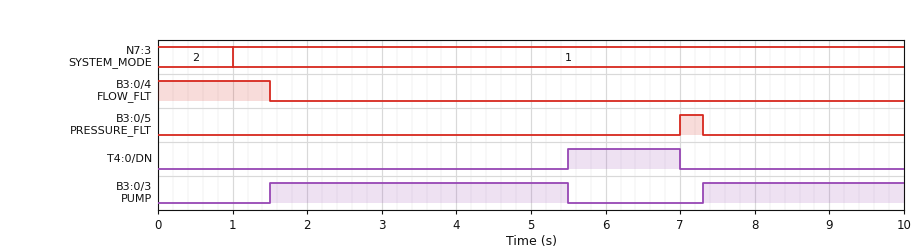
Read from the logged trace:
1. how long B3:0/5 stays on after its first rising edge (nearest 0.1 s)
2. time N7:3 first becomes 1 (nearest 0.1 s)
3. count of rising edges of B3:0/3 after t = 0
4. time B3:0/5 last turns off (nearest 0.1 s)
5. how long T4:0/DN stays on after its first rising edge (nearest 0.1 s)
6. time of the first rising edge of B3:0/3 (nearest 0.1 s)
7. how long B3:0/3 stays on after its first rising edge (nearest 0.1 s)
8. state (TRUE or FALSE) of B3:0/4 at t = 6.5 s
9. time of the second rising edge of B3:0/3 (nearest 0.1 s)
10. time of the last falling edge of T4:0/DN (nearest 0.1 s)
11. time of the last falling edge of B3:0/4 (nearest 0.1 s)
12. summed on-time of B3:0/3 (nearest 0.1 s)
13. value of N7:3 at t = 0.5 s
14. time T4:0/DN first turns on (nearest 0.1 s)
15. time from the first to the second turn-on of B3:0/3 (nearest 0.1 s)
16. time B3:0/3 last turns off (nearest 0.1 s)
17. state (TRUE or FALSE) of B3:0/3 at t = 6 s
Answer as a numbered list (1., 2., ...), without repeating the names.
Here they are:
1. 0.3 s
2. 1.0 s
3. 2
4. 7.3 s
5. 1.5 s
6. 1.5 s
7. 4.0 s
8. FALSE
9. 7.3 s
10. 7.0 s
11. 1.5 s
12. 6.7 s
13. 2
14. 5.5 s
15. 5.8 s
16. 5.5 s
17. FALSE
